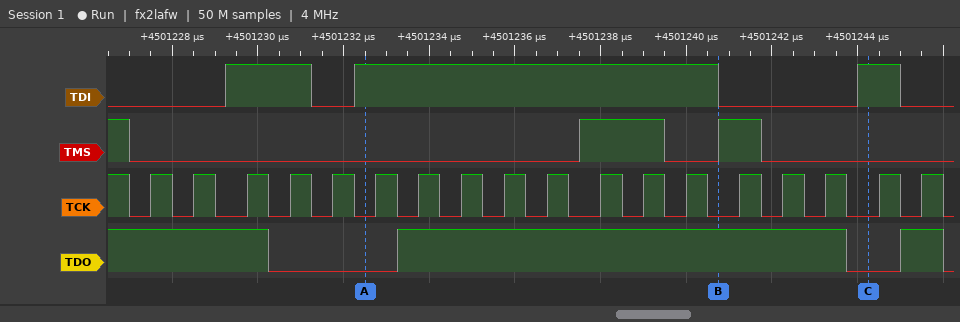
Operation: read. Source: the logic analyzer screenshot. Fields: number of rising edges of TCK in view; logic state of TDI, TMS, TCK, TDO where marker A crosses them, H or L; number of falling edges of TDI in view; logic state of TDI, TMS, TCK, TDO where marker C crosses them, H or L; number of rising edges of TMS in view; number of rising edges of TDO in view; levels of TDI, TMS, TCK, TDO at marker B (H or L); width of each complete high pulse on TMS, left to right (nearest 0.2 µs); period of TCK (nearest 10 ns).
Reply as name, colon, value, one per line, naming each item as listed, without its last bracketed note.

number of rising edges of TCK in view: 18
logic state of TDI, TMS, TCK, TDO where marker A crosses them, H or L: TDI=H, TMS=L, TCK=L, TDO=L
number of falling edges of TDI in view: 3
logic state of TDI, TMS, TCK, TDO where marker C crosses them, H or L: TDI=H, TMS=L, TCK=L, TDO=L
number of rising edges of TMS in view: 2
number of rising edges of TDO in view: 2
levels of TDI, TMS, TCK, TDO at marker B: TDI=L, TMS=H, TCK=L, TDO=H
width of each complete high pulse on TMS, left to right: 2 µs, 1 µs
period of TCK: 1060 ns
